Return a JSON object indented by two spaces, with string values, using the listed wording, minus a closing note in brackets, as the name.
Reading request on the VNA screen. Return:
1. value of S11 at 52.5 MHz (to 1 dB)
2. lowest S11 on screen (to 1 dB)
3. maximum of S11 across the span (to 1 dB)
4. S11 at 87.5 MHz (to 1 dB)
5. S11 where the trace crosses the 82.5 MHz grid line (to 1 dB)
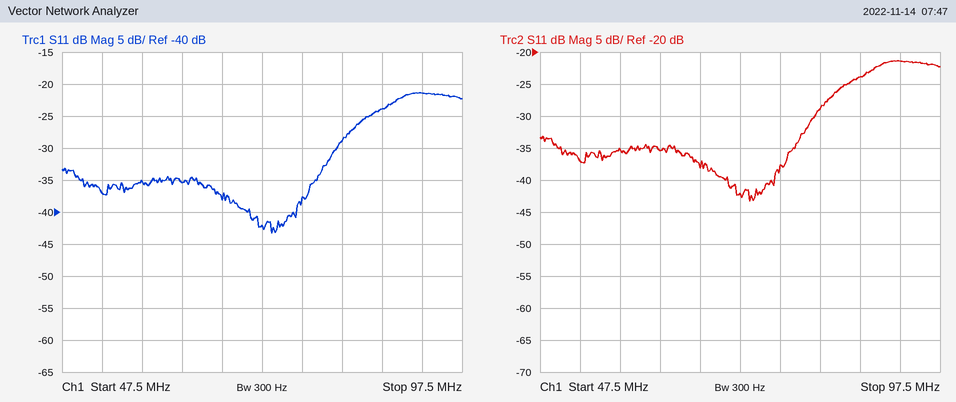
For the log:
{
  "value of S11 at 52.5 MHz": "-37 dB",
  "lowest S11 on screen": "-43 dB",
  "maximum of S11 across the span": "-21 dB",
  "S11 at 87.5 MHz": "-24 dB",
  "S11 where the trace crosses the 82.5 MHz grid line": "-29 dB"
}
